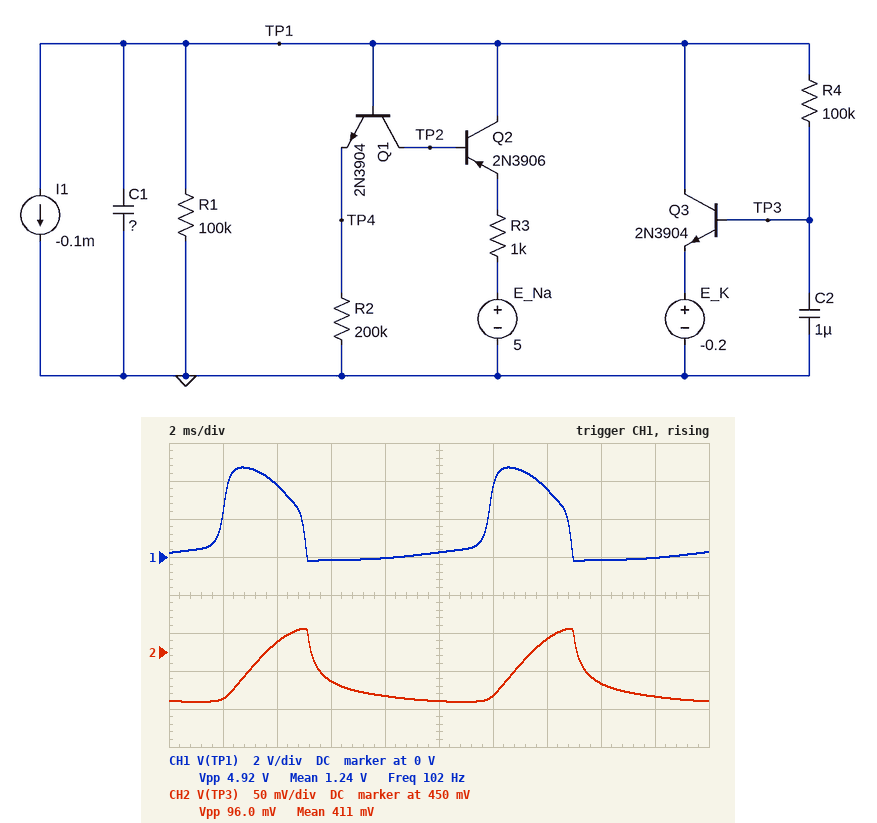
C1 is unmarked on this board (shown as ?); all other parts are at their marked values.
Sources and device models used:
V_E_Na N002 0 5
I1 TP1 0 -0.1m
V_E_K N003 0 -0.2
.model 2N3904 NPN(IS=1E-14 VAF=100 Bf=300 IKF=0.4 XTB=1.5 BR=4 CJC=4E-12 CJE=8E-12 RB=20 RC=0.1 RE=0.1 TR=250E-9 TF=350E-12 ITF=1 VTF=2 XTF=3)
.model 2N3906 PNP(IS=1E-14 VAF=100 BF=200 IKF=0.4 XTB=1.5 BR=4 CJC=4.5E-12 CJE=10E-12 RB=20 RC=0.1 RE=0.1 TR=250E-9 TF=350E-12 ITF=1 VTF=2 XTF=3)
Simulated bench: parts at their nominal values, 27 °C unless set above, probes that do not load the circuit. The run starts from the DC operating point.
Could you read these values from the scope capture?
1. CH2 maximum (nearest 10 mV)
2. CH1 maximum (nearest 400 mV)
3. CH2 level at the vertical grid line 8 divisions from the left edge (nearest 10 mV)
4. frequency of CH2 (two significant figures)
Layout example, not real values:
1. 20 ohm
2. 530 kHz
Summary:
1. 480 mV
2. 4.8 V
3. 410 mV
4. 100 Hz
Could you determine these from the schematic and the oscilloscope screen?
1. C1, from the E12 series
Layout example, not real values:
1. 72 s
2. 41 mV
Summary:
1. 180 nF
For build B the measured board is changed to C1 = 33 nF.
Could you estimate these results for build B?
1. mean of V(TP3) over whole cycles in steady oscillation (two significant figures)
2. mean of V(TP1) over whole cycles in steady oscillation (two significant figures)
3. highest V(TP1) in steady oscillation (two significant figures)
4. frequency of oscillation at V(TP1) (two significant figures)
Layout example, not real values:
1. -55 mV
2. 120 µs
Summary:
1. 420 mV
2. 1.5 V
3. 4.8 V
4. 150 Hz
